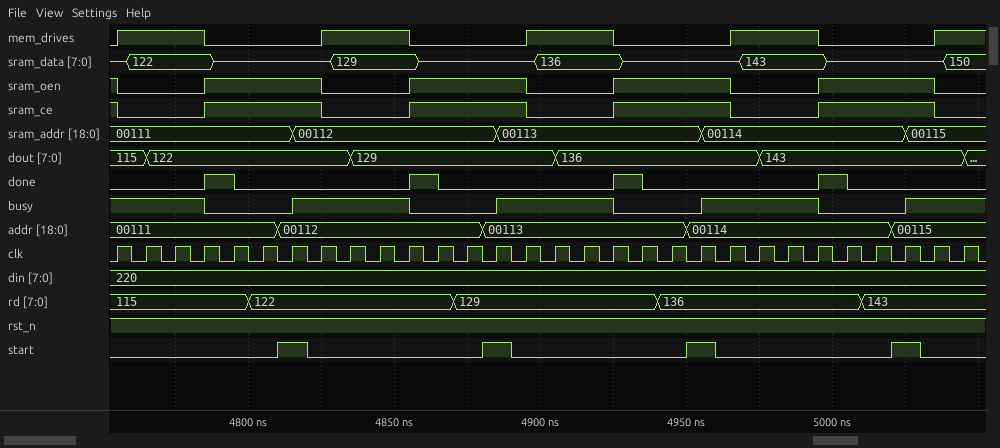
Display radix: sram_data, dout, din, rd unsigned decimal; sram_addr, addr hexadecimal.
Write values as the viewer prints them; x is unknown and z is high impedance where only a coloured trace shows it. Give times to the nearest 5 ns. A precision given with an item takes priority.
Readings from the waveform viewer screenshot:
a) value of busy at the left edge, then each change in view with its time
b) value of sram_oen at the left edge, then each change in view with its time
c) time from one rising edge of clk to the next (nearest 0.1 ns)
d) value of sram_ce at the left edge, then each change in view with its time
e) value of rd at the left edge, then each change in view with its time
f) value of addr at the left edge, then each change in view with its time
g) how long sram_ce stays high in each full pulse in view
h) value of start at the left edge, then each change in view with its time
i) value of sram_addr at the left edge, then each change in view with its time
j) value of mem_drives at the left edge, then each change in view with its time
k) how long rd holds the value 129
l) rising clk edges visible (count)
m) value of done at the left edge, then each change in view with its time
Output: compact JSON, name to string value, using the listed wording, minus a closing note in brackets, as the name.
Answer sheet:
{"value of busy at the left edge, then each change in view with its time": "1, 0 at 4785 ns, 1 at 4815 ns, 0 at 4855 ns, 1 at 4885 ns, 0 at 4925 ns, 1 at 4955 ns, 0 at 4995 ns, 1 at 5025 ns", "value of sram_oen at the left edge, then each change in view with its time": "1, 0 at 4755 ns, 1 at 4785 ns, 0 at 4825 ns, 1 at 4855 ns, 0 at 4895 ns, 1 at 4925 ns, 0 at 4965 ns, 1 at 4995 ns, 0 at 5035 ns", "time from one rising edge of clk to the next": "10 ns", "value of sram_ce at the left edge, then each change in view with its time": "1, 0 at 4755 ns, 1 at 4785 ns, 0 at 4825 ns, 1 at 4855 ns, 0 at 4895 ns, 1 at 4925 ns, 0 at 4965 ns, 1 at 4995 ns, 0 at 5035 ns", "value of rd at the left edge, then each change in view with its time": "115, 122 at 4800 ns, 129 at 4870 ns, 136 at 4940 ns, 143 at 5010 ns", "value of addr at the left edge, then each change in view with its time": "00111, 00112 at 4810 ns, 00113 at 4880 ns, 00114 at 4950 ns, 00115 at 5020 ns", "how long sram_ce stays high in each full pulse in view": "40 ns, 40 ns, 40 ns, 40 ns", "value of start at the left edge, then each change in view with its time": "0, 1 at 4810 ns, 0 at 4820 ns, 1 at 4880 ns, 0 at 4890 ns, 1 at 4950 ns, 0 at 4960 ns, 1 at 5020 ns, 0 at 5030 ns", "value of sram_addr at the left edge, then each change in view with its time": "00111, 00112 at 4815 ns, 00113 at 4885 ns, 00114 at 4955 ns, 00115 at 5025 ns", "value of mem_drives at the left edge, then each change in view with its time": "0, 1 at 4755 ns, 0 at 4785 ns, 1 at 4825 ns, 0 at 4855 ns, 1 at 4895 ns, 0 at 4925 ns, 1 at 4965 ns, 0 at 4995 ns, 1 at 5035 ns", "how long rd holds the value 129": "70 ns", "rising clk edges visible": "30", "value of done at the left edge, then each change in view with its time": "0, 1 at 4785 ns, 0 at 4795 ns, 1 at 4855 ns, 0 at 4865 ns, 1 at 4925 ns, 0 at 4935 ns, 1 at 4995 ns, 0 at 5005 ns"}
